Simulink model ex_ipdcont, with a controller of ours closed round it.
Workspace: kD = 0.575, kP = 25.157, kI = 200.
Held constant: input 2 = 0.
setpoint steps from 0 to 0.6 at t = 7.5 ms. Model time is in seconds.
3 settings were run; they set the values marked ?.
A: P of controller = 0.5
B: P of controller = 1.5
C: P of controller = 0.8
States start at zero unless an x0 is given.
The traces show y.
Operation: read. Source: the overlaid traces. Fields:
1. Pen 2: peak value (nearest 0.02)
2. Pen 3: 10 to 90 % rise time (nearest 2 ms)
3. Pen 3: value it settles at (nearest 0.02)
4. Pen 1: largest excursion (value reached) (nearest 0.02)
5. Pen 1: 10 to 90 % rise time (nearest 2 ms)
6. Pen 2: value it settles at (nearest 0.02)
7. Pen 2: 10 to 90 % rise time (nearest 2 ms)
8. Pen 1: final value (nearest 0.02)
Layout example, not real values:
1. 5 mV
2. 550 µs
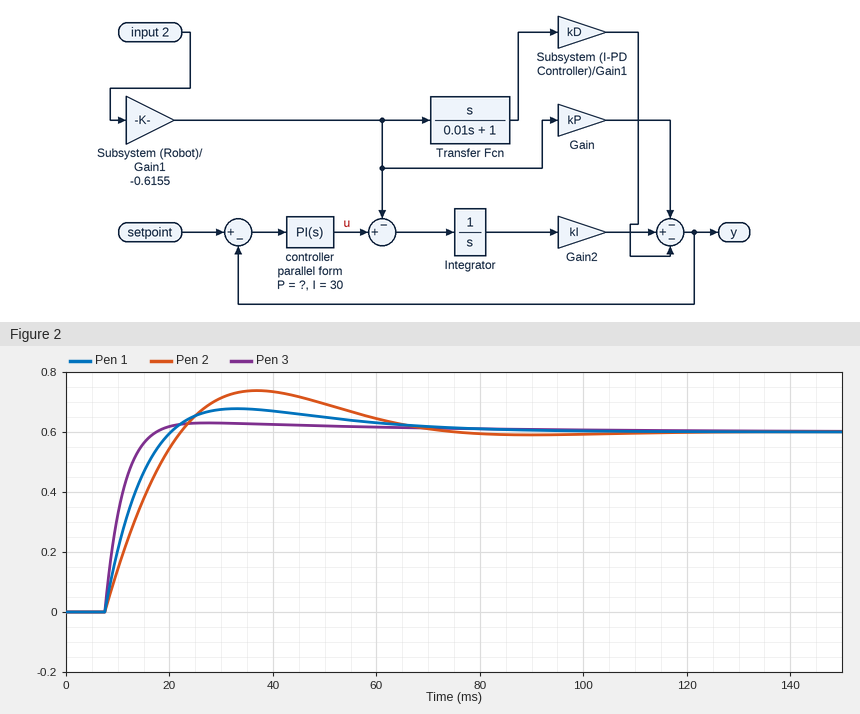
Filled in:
1. 0.74
2. 6 ms
3. 0.60
4. 0.68
5. 10 ms
6. 0.60
7. 12 ms
8. 0.60
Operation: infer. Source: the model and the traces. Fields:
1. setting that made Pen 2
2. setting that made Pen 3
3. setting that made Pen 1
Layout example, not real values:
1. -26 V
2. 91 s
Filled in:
1. A
2. B
3. C
